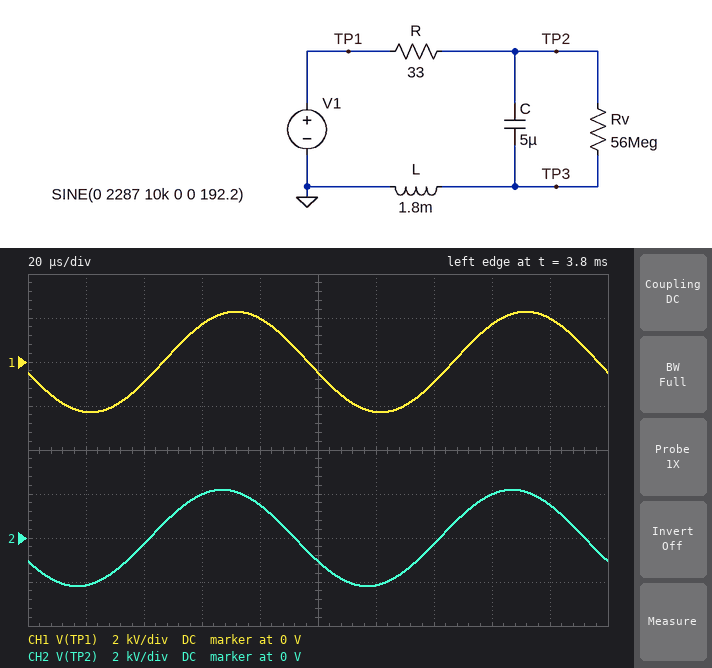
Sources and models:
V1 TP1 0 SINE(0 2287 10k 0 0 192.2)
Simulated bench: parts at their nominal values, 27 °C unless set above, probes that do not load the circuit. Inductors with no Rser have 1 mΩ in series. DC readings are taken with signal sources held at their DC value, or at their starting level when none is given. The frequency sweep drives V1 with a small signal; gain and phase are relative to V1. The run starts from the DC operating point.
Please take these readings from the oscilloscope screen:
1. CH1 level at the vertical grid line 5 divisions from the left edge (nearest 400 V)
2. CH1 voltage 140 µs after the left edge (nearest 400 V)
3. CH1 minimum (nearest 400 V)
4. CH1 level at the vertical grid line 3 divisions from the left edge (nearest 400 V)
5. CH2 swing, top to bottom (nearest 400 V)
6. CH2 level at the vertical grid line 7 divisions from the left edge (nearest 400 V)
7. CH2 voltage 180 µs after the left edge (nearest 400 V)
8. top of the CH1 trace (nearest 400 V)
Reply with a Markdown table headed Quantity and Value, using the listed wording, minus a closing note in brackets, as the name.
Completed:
| Quantity | Value |
|---|---|
| CH1 level at the vertical grid line 5 divisions from the left edge | -400 V |
| CH1 voltage 140 µs after the left edge | -800 V |
| CH1 minimum | -2.4 kV |
| CH1 level at the vertical grid line 3 divisions from the left edge | 1.6 kV |
| CH2 swing, top to bottom | 4.4 kV |
| CH2 level at the vertical grid line 7 divisions from the left edge | -400 V |
| CH2 voltage 180 µs after the left edge | 1.6 kV |
| top of the CH1 trace | 2.4 kV |
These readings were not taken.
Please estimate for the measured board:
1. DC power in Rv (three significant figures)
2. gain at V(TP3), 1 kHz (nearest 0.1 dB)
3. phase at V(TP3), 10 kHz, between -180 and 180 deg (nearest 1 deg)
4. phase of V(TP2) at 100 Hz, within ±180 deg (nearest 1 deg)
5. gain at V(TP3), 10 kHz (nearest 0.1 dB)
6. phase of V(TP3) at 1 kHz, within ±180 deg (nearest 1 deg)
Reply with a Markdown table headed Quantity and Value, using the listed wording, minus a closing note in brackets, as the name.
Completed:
| Quantity | Value |
|---|---|
| DC power in Rv | 4.17 mW |
| gain at V(TP3), 1 kHz | -10.7 dB |
| phase at V(TP3), 10 kHz, between -180 and 180 deg | 17 deg |
| phase of V(TP2) at 100 Hz, within ±180 deg | -6 deg |
| gain at V(TP3), 10 kHz | -0.1 dB |
| phase of V(TP3) at 1 kHz, within ±180 deg | 122 deg |
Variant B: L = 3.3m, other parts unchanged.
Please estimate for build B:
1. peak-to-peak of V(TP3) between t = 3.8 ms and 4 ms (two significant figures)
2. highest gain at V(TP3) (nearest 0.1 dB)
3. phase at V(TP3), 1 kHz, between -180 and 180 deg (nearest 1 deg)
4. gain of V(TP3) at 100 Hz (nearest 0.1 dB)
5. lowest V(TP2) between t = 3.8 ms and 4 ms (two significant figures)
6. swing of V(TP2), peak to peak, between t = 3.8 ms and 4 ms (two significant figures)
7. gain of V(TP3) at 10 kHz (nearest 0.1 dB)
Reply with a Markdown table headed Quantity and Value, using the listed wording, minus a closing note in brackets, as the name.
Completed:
| Quantity | Value |
|---|---|
| peak-to-peak of V(TP3) between t = 3.8 ms and 4 ms | 4.6 kV |
| highest gain at V(TP3) | 0.1 dB |
| phase at V(TP3), 1 kHz, between -180 and 180 deg | 109 deg |
| gain of V(TP3) at 100 Hz | -43.7 dB |
| lowest V(TP2) between t = 3.8 ms and 4 ms | -2.3 kV |
| swing of V(TP2), peak to peak, between t = 3.8 ms and 4 ms | 4.5 kV |
| gain of V(TP3) at 10 kHz | 0 dB |
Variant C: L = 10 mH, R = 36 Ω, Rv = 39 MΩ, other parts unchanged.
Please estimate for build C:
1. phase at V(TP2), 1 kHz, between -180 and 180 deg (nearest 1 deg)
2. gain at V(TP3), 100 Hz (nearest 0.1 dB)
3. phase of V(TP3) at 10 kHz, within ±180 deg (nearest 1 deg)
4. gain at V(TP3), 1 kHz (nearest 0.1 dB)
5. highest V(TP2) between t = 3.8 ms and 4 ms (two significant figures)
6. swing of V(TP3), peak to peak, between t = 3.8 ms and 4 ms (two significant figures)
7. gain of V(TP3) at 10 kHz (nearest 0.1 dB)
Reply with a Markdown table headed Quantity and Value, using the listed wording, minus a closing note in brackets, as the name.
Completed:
| Quantity | Value |
|---|---|
| phase at V(TP2), 1 kHz, between -180 and 180 deg | 49 deg |
| gain at V(TP3), 100 Hz | -34.0 dB |
| phase of V(TP3) at 10 kHz, within ±180 deg | 3 deg |
| gain at V(TP3), 1 kHz | 2.4 dB |
| highest V(TP2) between t = 3.8 ms and 4 ms | 2.3 kV |
| swing of V(TP3), peak to peak, between t = 3.8 ms and 4 ms | 4.6 kV |
| gain of V(TP3) at 10 kHz | 0 dB |
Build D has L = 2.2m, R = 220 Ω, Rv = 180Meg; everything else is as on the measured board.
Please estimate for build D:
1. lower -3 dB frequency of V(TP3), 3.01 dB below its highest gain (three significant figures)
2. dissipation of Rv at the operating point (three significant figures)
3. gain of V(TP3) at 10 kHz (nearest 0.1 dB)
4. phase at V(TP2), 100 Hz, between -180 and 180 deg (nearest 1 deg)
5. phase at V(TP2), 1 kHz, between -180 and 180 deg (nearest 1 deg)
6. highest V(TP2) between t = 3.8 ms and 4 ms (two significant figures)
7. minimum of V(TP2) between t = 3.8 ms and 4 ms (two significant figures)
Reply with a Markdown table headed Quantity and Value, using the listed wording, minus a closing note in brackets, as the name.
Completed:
| Quantity | Value |
|---|---|
| lower -3 dB frequency of V(TP3), 3.01 dB below its highest gain | 15.8 kHz |
| dissipation of Rv at the operating point | 1.30 mW |
| gain of V(TP3) at 10 kHz | -5.4 dB |
| phase at V(TP2), 100 Hz, between -180 and 180 deg | -35 deg |
| phase at V(TP2), 1 kHz, between -180 and 180 deg | -85 deg |
| highest V(TP2) between t = 3.8 ms and 4 ms | 1.2 kV |
| minimum of V(TP2) between t = 3.8 ms and 4 ms | -1.2 kV |
